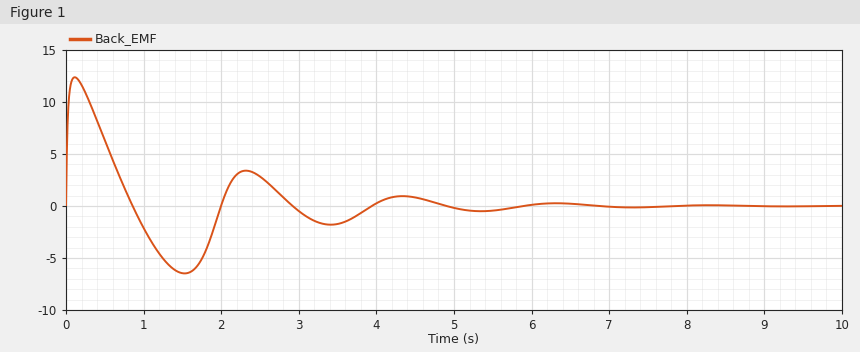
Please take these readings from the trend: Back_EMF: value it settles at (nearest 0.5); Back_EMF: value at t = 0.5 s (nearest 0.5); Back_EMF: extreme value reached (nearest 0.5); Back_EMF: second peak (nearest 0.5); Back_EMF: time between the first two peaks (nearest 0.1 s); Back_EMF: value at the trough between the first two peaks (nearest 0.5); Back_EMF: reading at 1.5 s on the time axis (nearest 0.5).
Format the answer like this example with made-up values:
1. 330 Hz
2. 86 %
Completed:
1. 0.0
2. 6.5
3. 12.5
4. 3.5
5. 2.2 s
6. -6.5
7. -6.5
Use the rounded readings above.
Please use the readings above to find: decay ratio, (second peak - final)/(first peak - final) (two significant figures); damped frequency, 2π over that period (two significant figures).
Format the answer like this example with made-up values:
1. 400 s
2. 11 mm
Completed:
1. 0.28
2. 2.9 rad/s
